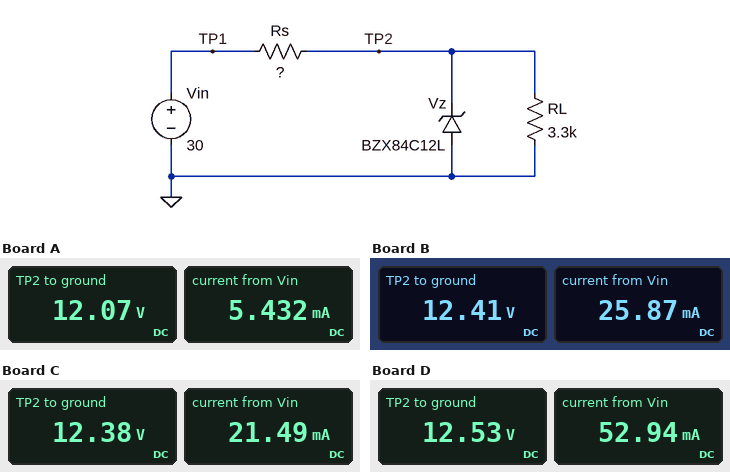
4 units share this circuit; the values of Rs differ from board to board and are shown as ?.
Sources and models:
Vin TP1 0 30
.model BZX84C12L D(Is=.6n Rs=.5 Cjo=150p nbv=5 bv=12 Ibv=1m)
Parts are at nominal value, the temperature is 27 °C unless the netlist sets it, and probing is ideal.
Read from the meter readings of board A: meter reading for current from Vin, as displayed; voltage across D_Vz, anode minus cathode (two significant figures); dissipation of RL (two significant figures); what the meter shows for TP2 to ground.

5.432 mA
-12 V
44 mW
12.07 V
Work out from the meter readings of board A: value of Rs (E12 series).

3.3 kΩ
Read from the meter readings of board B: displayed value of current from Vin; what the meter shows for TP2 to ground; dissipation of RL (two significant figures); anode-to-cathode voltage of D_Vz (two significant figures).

25.87 mA
12.41 V
47 mW
-12 V
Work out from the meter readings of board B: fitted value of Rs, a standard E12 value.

680 Ω
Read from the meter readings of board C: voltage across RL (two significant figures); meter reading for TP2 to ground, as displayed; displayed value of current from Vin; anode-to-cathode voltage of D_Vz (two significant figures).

12 V
12.38 V
21.49 mA
-12 V
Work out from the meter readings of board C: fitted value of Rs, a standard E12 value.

820 Ω
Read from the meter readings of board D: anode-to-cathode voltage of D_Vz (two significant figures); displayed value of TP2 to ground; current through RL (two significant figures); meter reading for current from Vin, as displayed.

-13 V
12.53 V
3.8 mA
52.94 mA
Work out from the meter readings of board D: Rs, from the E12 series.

330 Ω
